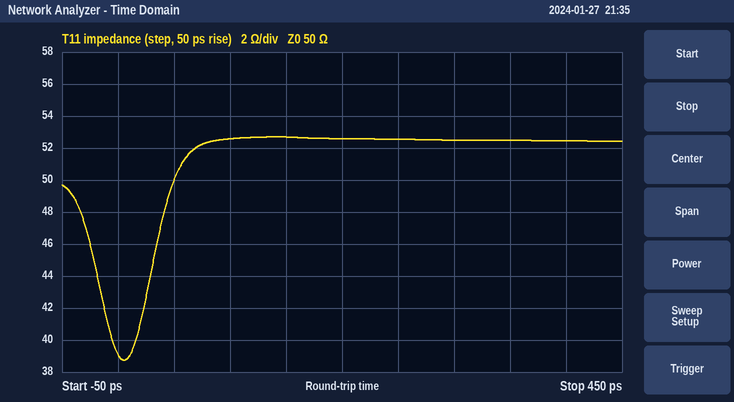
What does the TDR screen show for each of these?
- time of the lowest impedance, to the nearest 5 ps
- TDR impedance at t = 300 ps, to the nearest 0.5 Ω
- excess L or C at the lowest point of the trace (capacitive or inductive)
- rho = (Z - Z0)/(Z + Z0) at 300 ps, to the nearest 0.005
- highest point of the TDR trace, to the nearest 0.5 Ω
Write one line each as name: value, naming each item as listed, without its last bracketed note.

time of the lowest impedance, to the nearest 5 ps: 5 ps
TDR impedance at t = 300 ps, to the nearest 0.5 Ω: 52.5 Ω
excess L or C at the lowest point of the trace: capacitive
rho = (Z - Z0)/(Z + Z0) at 300 ps, to the nearest 0.005: +0.025
highest point of the TDR trace, to the nearest 0.5 Ω: 52.5 Ω
